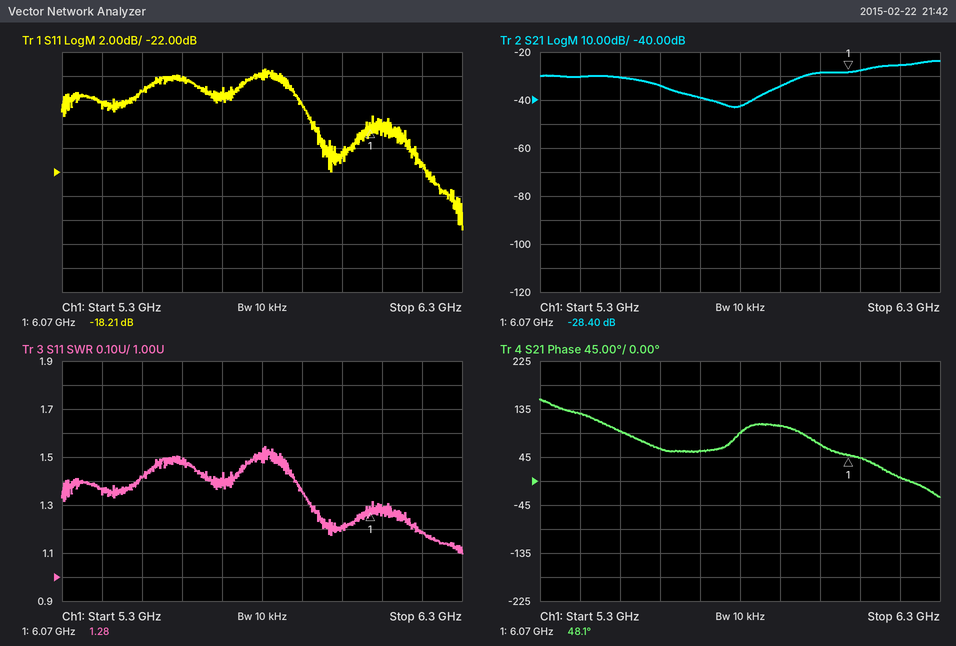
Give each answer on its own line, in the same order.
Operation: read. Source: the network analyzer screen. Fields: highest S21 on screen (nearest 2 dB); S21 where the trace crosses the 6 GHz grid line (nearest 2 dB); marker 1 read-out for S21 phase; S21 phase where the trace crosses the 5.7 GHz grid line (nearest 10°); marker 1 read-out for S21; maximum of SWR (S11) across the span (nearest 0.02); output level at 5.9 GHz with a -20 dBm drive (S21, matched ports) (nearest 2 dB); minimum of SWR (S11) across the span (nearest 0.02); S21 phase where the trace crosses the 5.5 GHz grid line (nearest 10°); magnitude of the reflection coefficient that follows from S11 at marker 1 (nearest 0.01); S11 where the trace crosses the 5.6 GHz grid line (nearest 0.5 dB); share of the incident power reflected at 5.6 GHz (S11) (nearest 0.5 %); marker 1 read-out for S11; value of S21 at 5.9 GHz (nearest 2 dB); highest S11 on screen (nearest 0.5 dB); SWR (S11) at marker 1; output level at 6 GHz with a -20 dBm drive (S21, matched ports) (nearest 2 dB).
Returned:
-24 dB
-28 dB
48.1°
60°
-28.40 dB
1.54
-54 dBm
1.10
90°
0.12
-14.0 dB
4.0 %
-18.21 dB
-34 dB
-13.5 dB
1.28
-48 dBm
